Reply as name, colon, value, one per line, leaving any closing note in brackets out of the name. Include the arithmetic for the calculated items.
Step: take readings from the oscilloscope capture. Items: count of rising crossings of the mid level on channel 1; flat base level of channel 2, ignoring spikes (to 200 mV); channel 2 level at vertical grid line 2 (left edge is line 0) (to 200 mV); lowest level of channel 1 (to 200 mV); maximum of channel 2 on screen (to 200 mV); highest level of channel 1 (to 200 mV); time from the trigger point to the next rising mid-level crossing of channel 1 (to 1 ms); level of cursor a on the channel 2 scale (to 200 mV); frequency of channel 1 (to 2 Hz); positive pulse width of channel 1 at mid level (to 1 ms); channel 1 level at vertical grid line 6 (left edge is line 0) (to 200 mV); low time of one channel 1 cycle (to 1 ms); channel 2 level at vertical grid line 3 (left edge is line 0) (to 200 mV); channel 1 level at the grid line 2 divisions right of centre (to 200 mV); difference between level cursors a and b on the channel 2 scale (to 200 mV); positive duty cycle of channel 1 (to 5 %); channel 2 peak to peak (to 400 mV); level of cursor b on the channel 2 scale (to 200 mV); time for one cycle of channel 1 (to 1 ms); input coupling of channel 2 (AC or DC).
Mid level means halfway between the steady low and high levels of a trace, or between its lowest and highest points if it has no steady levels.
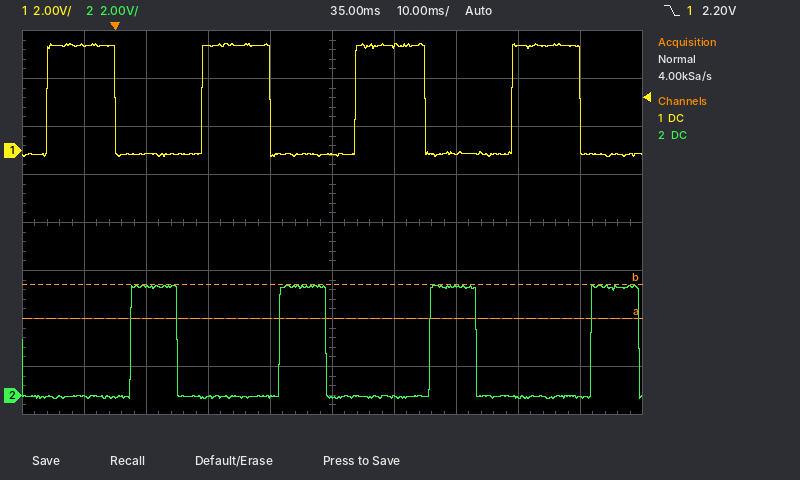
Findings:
count of rising crossings of the mid level on channel 1: 4
flat base level of channel 2, ignoring spikes: 0.0 V
channel 2 level at vertical grid line 2 (left edge is line 0): 4.6 V
lowest level of channel 1: -200 mV
maximum of channel 2 on screen: 4.6 V
highest level of channel 1: 4.4 V
time from the trigger point to the next rising mid-level crossing of channel 1: 14 ms
level of cursor a on the channel 2 scale: 3.2 V
frequency of channel 1: 1 / 25 ms ≈ 40 Hz
positive pulse width of channel 1 at mid level: 11 ms
channel 1 level at vertical grid line 6 (left edge is line 0): 4.4 V
low time of one channel 1 cycle: 14 ms
channel 2 level at vertical grid line 3 (left edge is line 0): 0.0 V
channel 1 level at the grid line 2 divisions right of centre: -200 mV
difference between level cursors a and b on the channel 2 scale: 1.4 V
positive duty cycle of channel 1: 11 ms / 25 ms ≈ 44.0 %, so 45 % to the nearest 5 %
channel 2 peak to peak: 4.8 V
level of cursor b on the channel 2 scale: 4.6 V
time for one cycle of channel 1: 25 ms
input coupling of channel 2: DC
